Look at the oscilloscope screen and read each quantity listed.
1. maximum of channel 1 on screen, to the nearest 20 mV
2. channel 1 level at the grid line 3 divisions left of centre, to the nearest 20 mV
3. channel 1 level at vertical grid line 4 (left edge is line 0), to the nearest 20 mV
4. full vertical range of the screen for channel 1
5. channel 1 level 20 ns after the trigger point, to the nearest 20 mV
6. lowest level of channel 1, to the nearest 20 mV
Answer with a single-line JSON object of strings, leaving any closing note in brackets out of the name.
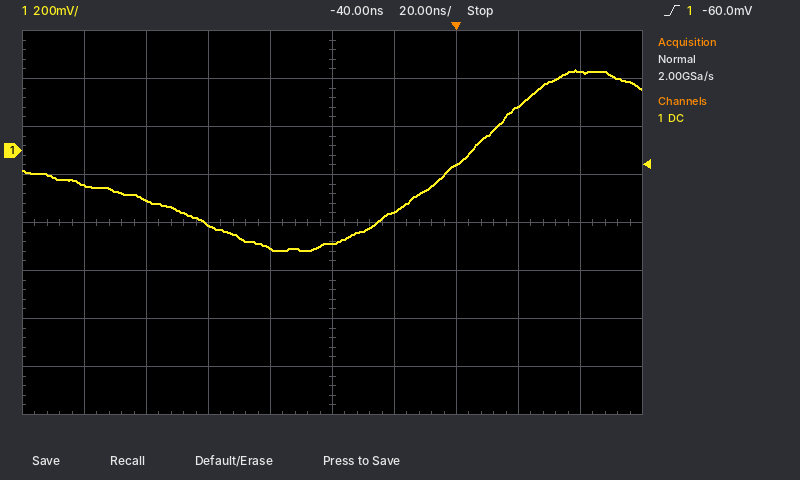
{"maximum of channel 1 on screen, to the nearest 20 mV": "340 mV", "channel 1 level at the grid line 3 divisions left of centre, to the nearest 20 mV": "-200 mV", "channel 1 level at vertical grid line 4 (left edge is line 0), to the nearest 20 mV": "-400 mV", "full vertical range of the screen for channel 1": "1.6 V", "channel 1 level 20 ns after the trigger point, to the nearest 20 mV": "180 mV", "lowest level of channel 1, to the nearest 20 mV": "-420 mV"}
